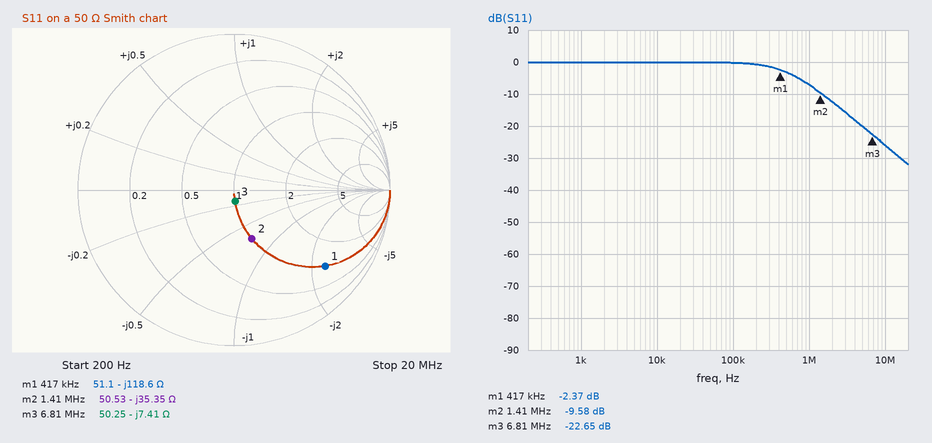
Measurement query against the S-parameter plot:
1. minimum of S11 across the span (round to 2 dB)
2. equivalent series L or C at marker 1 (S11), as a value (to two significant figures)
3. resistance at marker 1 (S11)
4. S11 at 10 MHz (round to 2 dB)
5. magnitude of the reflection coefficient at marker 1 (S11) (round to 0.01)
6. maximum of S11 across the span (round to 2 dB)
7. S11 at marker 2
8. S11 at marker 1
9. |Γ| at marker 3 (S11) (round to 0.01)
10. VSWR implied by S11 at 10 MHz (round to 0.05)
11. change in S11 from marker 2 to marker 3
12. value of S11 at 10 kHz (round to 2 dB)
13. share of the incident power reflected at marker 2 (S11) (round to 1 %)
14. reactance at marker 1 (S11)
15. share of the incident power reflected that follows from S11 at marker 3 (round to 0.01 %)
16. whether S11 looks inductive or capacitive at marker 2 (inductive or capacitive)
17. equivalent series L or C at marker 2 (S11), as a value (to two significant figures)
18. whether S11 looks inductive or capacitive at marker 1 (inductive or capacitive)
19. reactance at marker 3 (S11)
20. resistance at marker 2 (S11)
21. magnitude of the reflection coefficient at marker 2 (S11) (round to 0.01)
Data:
-32 dB
3.2 nF
51.1 Ω
-26 dB
0.76
0 dB
-9.58 dB
-2.37 dB
0.07
1.10
-13.07 dB
0 dB
11 %
-118.6 Ω
0.54 %
capacitive
3.2 nF
capacitive
-7.41 Ω
50.53 Ω
0.33
